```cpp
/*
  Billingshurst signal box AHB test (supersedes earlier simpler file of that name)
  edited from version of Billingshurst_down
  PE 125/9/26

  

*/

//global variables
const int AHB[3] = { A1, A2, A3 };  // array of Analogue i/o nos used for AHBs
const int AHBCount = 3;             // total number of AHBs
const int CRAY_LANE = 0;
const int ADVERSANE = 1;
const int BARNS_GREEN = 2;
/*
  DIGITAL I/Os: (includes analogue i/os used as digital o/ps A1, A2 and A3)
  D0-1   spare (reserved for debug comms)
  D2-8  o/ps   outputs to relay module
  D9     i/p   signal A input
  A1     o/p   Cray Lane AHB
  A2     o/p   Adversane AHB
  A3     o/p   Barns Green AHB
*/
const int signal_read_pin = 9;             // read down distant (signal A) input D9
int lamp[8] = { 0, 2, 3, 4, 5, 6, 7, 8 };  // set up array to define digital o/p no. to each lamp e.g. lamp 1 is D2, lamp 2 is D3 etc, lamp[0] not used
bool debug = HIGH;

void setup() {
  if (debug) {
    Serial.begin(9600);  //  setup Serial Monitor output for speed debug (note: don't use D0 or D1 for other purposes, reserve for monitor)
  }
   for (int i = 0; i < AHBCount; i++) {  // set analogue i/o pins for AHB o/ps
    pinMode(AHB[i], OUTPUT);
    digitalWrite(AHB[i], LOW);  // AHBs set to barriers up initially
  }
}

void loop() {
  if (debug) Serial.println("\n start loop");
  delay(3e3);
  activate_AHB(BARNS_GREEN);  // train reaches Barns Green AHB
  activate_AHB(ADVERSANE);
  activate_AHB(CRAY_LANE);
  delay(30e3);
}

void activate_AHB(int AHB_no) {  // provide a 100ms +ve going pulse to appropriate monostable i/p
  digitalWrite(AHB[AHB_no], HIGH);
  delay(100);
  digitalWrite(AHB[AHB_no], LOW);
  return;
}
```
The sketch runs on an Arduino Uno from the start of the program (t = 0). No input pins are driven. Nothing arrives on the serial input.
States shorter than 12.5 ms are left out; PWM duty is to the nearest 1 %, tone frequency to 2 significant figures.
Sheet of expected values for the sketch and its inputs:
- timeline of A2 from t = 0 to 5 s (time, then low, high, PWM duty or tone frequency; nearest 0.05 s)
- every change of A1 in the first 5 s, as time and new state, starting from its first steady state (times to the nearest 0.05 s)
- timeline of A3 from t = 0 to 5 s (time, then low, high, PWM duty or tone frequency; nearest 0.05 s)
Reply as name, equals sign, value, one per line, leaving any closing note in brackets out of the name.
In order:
timeline of A2 from t = 0 to 5 s = 0 s low; 3.1 s high; 3.2 s low
every change of A1 in the first 5 s, as time and new state, starting from its first steady state = 0 s low; 3.2 s high; 3.3 s low
timeline of A3 from t = 0 to 5 s = 0 s low; 3 s high; 3.1 s low
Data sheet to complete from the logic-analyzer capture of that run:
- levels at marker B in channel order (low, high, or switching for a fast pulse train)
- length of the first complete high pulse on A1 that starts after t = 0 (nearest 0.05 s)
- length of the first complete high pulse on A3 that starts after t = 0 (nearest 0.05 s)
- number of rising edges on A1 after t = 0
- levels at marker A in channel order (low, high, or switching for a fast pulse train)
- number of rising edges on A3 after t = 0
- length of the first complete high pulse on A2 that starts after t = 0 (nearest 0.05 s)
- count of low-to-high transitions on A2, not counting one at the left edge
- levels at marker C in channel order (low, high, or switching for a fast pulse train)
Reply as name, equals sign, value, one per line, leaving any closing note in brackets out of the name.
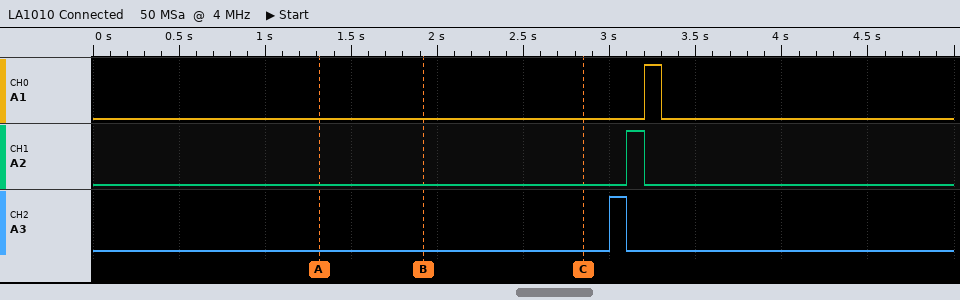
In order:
levels at marker B in channel order = A1 low, A2 low, A3 low
length of the first complete high pulse on A1 that starts after t = 0 = 0.10 s
length of the first complete high pulse on A3 that starts after t = 0 = 0.10 s
number of rising edges on A1 after t = 0 = 1
levels at marker A in channel order = A1 low, A2 low, A3 low
number of rising edges on A3 after t = 0 = 1
length of the first complete high pulse on A2 that starts after t = 0 = 0.10 s
count of low-to-high transitions on A2, not counting one at the left edge = 1
levels at marker C in channel order = A1 low, A2 low, A3 low
